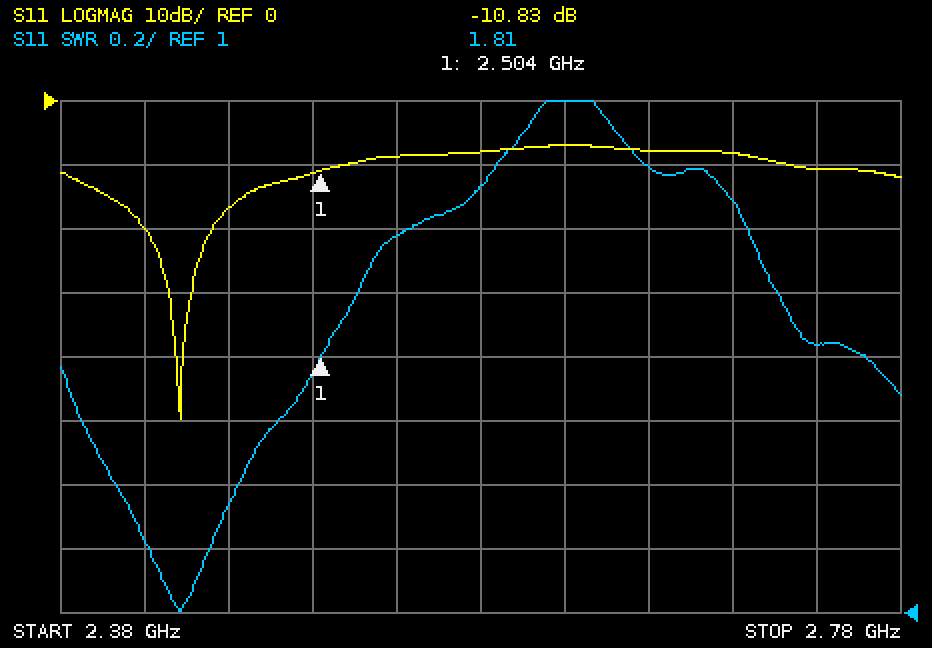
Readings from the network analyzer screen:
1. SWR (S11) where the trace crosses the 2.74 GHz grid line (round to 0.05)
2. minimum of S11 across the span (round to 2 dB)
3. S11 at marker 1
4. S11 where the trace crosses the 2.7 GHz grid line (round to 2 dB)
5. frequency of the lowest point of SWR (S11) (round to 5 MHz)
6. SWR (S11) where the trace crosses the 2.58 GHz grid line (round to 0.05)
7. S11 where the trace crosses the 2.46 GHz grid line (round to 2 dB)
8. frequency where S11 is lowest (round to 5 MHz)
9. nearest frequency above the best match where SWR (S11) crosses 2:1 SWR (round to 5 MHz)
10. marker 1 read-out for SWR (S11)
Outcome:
1.85
-50 dB
-10.83 dB
-8 dB
2.435 GHz
2.35
-16 dB
2.435 GHz
2.520 GHz
1.81
